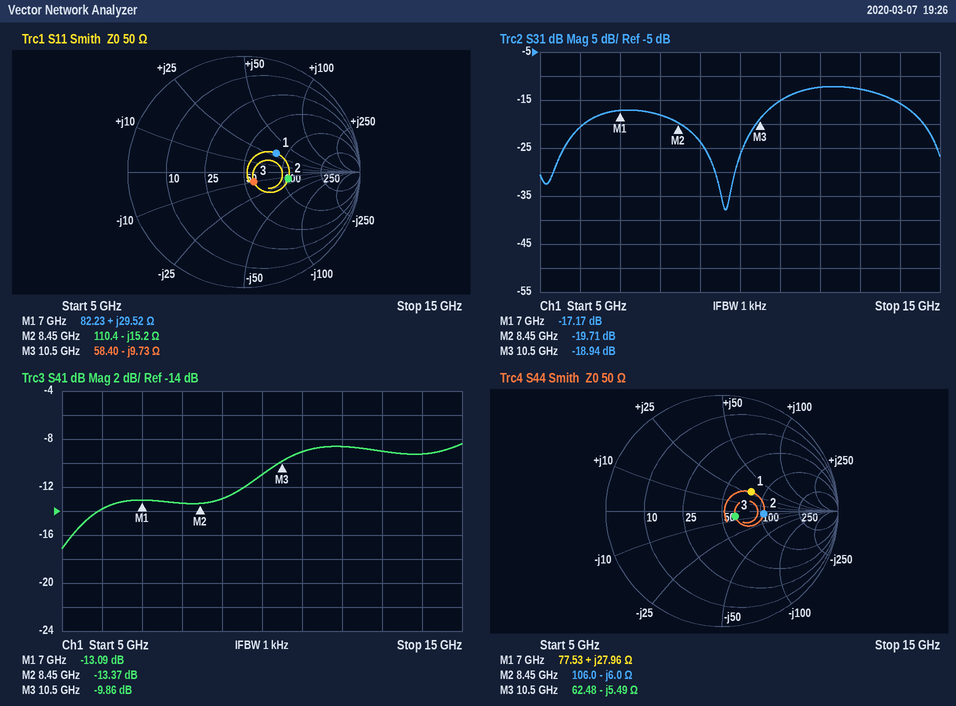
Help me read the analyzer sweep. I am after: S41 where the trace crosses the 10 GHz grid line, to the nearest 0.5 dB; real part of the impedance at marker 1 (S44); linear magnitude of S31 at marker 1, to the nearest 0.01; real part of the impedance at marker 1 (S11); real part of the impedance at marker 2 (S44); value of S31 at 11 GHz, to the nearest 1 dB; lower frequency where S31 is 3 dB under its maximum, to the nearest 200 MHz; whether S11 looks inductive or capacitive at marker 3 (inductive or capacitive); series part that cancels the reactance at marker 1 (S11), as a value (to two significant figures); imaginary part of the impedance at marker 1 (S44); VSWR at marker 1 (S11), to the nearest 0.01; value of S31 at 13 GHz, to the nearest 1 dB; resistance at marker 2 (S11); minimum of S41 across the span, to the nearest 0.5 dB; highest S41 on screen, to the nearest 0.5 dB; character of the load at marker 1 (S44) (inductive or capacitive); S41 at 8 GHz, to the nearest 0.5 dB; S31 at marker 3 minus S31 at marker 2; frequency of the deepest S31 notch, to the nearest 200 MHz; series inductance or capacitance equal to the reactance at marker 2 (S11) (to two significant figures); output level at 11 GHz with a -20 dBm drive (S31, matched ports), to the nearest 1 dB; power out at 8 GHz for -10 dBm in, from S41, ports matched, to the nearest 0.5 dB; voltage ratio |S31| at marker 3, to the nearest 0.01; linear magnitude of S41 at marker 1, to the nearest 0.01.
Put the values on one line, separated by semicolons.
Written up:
-11.0 dB; 77.53 Ω; 0.14; 82.23 Ω; 106.0 Ω; -15 dB; 11.0 GHz; capacitive; 770 fF; +27.96 Ω; 1.95; -13 dB; 110.4 Ω; -17.0 dB; -8.5 dB; inductive; -13.5 dB; 0.77 dB; 9.6 GHz; 1.2 pF; -35 dBm; -23.5 dBm; 0.11; 0.22
